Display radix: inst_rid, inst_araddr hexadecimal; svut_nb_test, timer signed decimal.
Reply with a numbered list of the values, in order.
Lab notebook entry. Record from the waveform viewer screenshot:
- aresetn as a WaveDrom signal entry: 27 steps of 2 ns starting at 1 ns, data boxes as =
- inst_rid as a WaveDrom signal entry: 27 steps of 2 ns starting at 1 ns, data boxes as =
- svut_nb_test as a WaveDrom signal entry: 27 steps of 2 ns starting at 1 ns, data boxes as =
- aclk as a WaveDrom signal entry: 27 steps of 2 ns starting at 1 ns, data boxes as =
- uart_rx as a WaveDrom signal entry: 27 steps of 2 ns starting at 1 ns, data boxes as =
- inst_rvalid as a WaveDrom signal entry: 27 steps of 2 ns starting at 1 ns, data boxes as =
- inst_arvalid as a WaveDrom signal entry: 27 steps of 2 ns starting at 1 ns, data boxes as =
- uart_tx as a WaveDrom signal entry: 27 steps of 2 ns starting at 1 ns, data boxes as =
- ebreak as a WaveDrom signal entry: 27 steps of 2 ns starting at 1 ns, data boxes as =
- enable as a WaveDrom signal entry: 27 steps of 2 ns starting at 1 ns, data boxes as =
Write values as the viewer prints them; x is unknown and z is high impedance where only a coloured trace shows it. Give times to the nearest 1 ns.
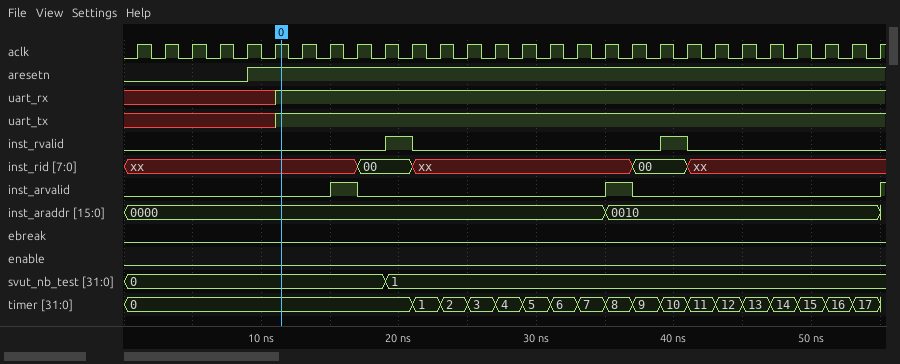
1. {name: 'aresetn', wave: '0...1......................'}
2. {name: 'inst_rid', wave: 'x.......=.x.......=.x......', data: '00 00'}
3. {name: 'svut_nb_test', wave: '=........=.................', data: '0 1'}
4. {name: 'aclk', wave: 'p..........................'}
5. {name: 'uart_rx', wave: 'x....1.....................'}
6. {name: 'inst_rvalid', wave: '0........10........10......'}
7. {name: 'inst_arvalid', wave: '0......10........10........'}
8. {name: 'uart_tx', wave: 'x....1.....................'}
9. {name: 'ebreak', wave: '0..........................'}
10. {name: 'enable', wave: '0..........................'}
